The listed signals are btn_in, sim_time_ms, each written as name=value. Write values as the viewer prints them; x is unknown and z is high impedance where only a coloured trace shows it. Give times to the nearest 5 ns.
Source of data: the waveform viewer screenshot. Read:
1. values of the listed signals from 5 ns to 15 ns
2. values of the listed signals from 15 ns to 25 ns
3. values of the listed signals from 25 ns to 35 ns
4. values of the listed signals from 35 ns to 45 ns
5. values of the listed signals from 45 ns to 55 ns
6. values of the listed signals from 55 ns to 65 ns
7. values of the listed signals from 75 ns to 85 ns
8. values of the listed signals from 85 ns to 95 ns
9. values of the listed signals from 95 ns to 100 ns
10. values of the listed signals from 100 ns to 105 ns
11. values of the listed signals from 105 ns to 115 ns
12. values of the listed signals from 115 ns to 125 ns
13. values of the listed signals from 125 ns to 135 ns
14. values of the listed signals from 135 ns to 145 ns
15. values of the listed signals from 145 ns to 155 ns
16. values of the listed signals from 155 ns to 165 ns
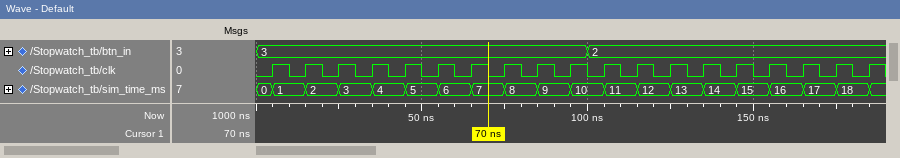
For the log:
btn_in=3, sim_time_ms=1
btn_in=3, sim_time_ms=2
btn_in=3, sim_time_ms=3
btn_in=3, sim_time_ms=4
btn_in=3, sim_time_ms=5
btn_in=3, sim_time_ms=6
btn_in=3, sim_time_ms=8
btn_in=3, sim_time_ms=9
btn_in=3, sim_time_ms=10
btn_in=2, sim_time_ms=10
btn_in=2, sim_time_ms=11
btn_in=2, sim_time_ms=12
btn_in=2, sim_time_ms=13
btn_in=2, sim_time_ms=14
btn_in=2, sim_time_ms=15
btn_in=2, sim_time_ms=16
